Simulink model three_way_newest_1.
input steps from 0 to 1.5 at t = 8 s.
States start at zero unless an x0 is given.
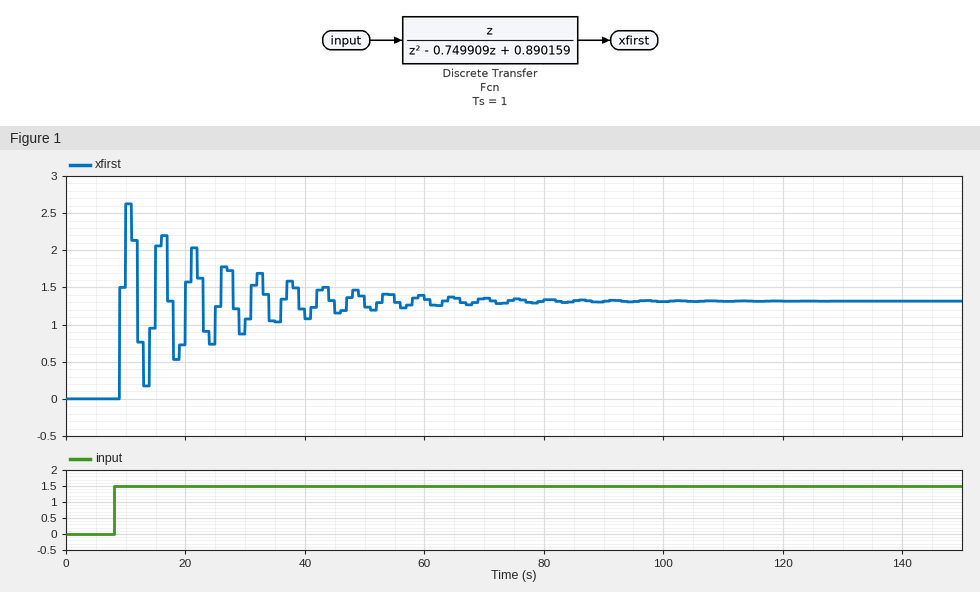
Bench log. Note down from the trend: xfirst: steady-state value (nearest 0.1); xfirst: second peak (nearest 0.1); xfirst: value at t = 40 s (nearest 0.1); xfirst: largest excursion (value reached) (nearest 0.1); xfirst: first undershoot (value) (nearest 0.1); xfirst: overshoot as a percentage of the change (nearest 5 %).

1.3
2.2
1.1
2.6
0.2
100 %
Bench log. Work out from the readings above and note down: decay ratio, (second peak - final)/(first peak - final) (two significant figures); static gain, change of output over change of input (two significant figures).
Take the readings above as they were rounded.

0.69
0.87
